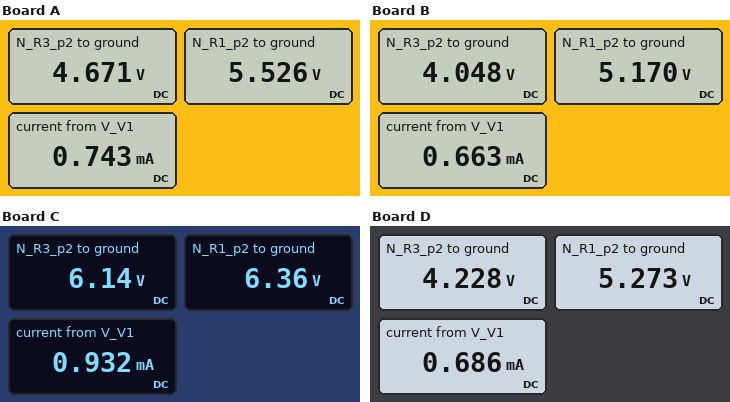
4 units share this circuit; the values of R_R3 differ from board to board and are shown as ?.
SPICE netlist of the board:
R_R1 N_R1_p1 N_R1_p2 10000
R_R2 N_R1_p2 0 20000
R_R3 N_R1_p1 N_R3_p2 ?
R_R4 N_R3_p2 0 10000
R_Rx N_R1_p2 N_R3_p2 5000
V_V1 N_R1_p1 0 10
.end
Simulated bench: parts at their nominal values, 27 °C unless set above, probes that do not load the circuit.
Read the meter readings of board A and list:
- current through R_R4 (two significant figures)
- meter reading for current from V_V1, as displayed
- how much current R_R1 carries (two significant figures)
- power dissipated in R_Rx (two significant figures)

470 µA
0.743 mA
450 µA
150 µW
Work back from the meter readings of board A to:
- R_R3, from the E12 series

18 kΩ
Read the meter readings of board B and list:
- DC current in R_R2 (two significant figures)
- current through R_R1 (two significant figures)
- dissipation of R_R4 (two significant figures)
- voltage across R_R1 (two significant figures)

260 µA
480 µA
1.6 mW
4.8 V
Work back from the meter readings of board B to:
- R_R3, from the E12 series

33 kΩ
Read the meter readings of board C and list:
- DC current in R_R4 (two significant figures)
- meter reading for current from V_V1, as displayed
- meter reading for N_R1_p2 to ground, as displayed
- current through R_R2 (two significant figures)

610 µA
0.932 mA
6.36 V
320 µA
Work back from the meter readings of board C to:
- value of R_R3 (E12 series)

6.8 kΩ
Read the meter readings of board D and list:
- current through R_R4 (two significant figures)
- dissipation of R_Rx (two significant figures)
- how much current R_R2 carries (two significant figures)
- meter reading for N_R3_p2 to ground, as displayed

420 µA
220 µW
260 µA
4.228 V
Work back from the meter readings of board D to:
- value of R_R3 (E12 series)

27 kΩ
